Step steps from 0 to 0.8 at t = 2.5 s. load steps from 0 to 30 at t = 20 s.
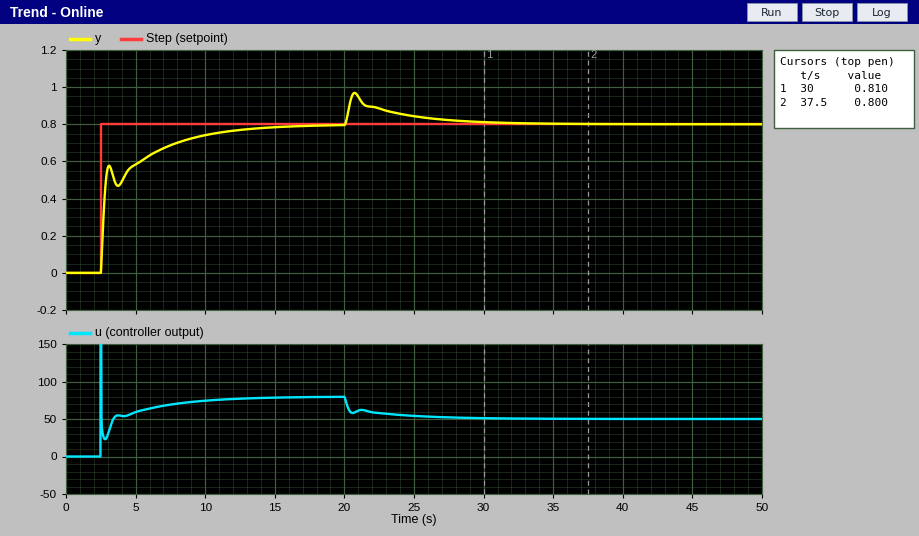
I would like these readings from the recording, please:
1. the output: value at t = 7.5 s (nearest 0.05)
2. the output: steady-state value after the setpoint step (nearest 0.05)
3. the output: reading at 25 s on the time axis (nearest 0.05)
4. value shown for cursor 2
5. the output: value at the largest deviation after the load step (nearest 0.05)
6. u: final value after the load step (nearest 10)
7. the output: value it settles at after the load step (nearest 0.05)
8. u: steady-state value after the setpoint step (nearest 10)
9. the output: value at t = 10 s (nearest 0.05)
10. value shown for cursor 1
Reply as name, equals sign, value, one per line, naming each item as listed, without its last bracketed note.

the output: value at t = 7.5 s = 0.70
the output: steady-state value after the setpoint step = 0.80
the output: reading at 25 s on the time axis = 0.85
value shown for cursor 2 = 0.800
the output: value at the largest deviation after the load step = 0.95
u: final value after the load step = 50
the output: value it settles at after the load step = 0.80
u: steady-state value after the setpoint step = 80
the output: value at t = 10 s = 0.75
value shown for cursor 1 = 0.810
